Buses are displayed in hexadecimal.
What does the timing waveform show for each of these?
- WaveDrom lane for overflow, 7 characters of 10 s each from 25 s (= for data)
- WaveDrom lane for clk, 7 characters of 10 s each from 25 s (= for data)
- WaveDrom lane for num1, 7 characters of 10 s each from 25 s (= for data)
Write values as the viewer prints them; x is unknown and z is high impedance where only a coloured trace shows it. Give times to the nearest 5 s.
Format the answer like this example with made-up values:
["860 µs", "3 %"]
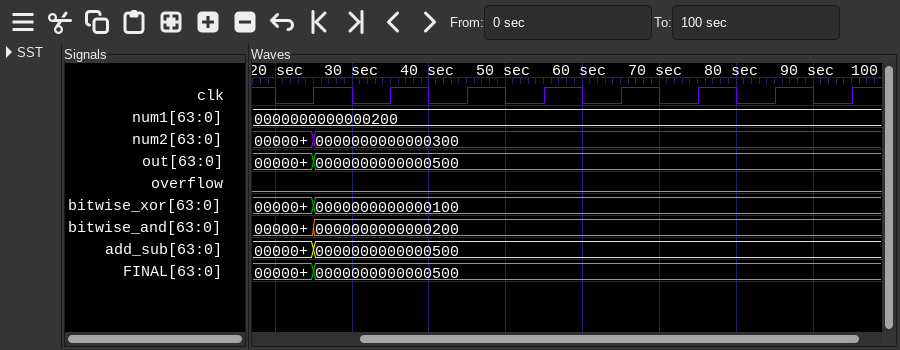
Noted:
["{name: 'overflow', wave: '0......'}", "{name: 'clk', wave: 'p......'}", "{name: 'num1', wave: '=......', data: '0000000000000200'}"]
